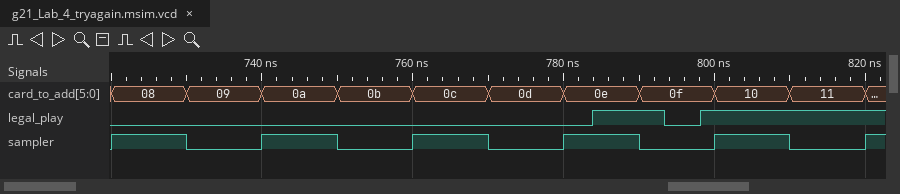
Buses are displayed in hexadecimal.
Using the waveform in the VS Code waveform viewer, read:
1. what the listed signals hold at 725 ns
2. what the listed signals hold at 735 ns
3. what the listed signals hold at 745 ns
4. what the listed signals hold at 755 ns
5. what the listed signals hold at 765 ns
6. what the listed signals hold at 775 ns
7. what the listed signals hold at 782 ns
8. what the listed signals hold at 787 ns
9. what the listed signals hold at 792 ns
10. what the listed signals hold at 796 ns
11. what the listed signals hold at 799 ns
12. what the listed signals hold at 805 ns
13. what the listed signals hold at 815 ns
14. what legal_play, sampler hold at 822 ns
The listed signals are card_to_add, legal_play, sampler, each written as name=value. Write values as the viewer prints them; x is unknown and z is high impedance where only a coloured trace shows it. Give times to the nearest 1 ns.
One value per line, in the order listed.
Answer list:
card_to_add=08, legal_play=0, sampler=1
card_to_add=09, legal_play=0, sampler=0
card_to_add=0a, legal_play=0, sampler=1
card_to_add=0b, legal_play=0, sampler=0
card_to_add=0c, legal_play=0, sampler=1
card_to_add=0d, legal_play=0, sampler=0
card_to_add=0e, legal_play=0, sampler=1
card_to_add=0e, legal_play=1, sampler=1
card_to_add=0f, legal_play=1, sampler=0
card_to_add=0f, legal_play=0, sampler=0
card_to_add=0f, legal_play=1, sampler=0
card_to_add=10, legal_play=1, sampler=1
card_to_add=11, legal_play=1, sampler=0
legal_play=1, sampler=1
